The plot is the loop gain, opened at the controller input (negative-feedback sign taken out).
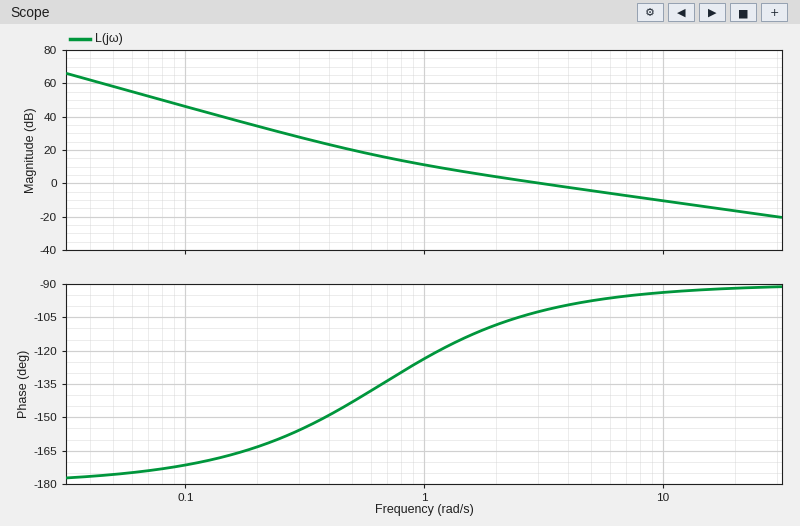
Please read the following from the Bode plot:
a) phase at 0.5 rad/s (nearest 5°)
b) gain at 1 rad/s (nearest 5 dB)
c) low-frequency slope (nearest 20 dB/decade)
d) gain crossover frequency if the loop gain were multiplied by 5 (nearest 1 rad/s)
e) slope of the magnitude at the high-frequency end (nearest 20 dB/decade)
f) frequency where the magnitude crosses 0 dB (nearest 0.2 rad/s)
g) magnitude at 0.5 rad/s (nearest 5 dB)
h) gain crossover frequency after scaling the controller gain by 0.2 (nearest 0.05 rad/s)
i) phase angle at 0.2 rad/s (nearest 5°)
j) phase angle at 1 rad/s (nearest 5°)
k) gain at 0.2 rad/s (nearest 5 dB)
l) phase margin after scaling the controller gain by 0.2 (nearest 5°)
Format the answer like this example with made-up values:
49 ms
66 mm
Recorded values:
-145°
10 dB
-40 dB/decade
15 rad/s
-20 dB/decade
3.0 rad/s
20 dB
0.80 rad/s
-165°
-125°
35 dB
50°
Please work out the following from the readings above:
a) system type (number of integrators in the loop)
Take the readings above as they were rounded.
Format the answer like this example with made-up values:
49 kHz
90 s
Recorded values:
2
